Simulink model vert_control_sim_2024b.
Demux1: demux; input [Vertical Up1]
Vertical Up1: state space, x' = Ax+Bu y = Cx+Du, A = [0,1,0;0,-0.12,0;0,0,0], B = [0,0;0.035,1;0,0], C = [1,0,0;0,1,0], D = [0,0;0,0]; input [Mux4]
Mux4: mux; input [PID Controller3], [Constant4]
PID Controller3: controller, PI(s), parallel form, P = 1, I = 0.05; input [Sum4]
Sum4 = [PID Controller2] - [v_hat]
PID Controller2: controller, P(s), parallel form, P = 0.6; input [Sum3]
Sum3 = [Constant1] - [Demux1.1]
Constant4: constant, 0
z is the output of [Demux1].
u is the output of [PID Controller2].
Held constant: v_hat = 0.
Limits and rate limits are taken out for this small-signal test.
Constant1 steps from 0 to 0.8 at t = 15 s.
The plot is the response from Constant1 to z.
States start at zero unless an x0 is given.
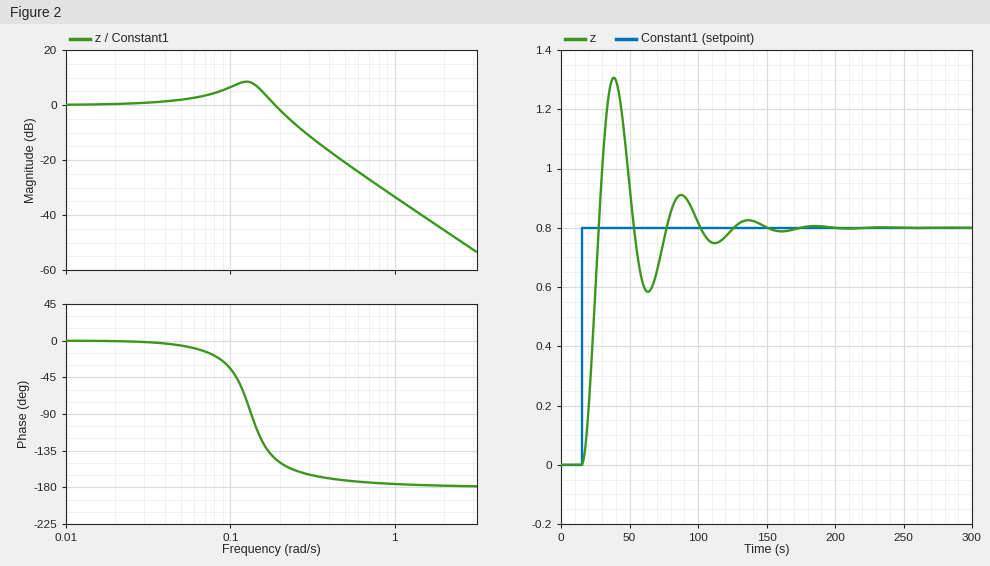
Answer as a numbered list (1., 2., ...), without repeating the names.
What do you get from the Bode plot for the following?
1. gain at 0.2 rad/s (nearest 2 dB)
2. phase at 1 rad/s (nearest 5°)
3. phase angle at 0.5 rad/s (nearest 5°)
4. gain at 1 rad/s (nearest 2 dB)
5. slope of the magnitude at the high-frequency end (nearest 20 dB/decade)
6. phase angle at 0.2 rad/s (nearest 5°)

1. -2 dB
2. -175°
3. -170°
4. -34 dB
5. -40 dB/decade
6. -150°
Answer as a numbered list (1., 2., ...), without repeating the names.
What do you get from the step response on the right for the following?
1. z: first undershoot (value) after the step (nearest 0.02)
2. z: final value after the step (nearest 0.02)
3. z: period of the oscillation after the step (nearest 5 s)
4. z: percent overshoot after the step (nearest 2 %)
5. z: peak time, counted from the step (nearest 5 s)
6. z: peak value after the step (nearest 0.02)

1. 0.58
2. 0.80
3. 50 s
4. 64 %
5. 25 s
6. 1.30
